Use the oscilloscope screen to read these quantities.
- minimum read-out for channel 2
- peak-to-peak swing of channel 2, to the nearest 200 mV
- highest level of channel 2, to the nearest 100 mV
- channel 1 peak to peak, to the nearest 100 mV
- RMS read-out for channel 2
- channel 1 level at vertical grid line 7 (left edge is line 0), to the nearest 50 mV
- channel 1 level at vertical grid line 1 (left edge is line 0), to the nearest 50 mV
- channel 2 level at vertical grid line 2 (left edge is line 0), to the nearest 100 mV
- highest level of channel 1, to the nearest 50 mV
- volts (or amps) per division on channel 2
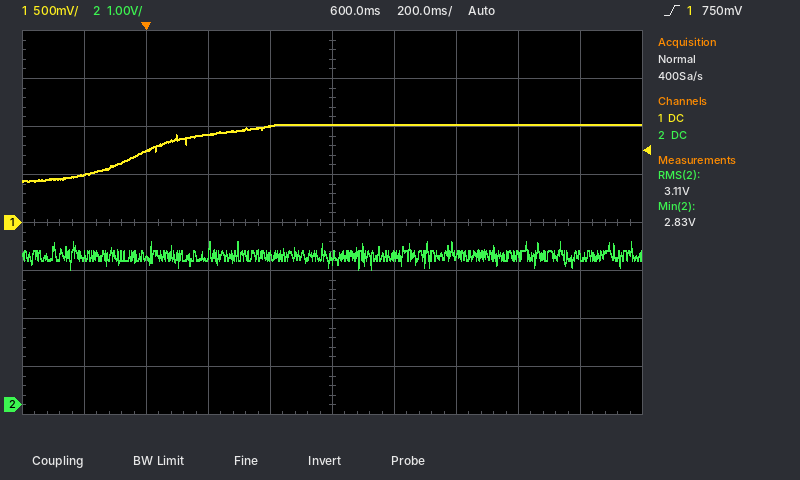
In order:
2.83 V
600 mV
3.4 V
600 mV
3.11 V
1.00 V
500 mV
3.1 V
1.00 V
1 V
